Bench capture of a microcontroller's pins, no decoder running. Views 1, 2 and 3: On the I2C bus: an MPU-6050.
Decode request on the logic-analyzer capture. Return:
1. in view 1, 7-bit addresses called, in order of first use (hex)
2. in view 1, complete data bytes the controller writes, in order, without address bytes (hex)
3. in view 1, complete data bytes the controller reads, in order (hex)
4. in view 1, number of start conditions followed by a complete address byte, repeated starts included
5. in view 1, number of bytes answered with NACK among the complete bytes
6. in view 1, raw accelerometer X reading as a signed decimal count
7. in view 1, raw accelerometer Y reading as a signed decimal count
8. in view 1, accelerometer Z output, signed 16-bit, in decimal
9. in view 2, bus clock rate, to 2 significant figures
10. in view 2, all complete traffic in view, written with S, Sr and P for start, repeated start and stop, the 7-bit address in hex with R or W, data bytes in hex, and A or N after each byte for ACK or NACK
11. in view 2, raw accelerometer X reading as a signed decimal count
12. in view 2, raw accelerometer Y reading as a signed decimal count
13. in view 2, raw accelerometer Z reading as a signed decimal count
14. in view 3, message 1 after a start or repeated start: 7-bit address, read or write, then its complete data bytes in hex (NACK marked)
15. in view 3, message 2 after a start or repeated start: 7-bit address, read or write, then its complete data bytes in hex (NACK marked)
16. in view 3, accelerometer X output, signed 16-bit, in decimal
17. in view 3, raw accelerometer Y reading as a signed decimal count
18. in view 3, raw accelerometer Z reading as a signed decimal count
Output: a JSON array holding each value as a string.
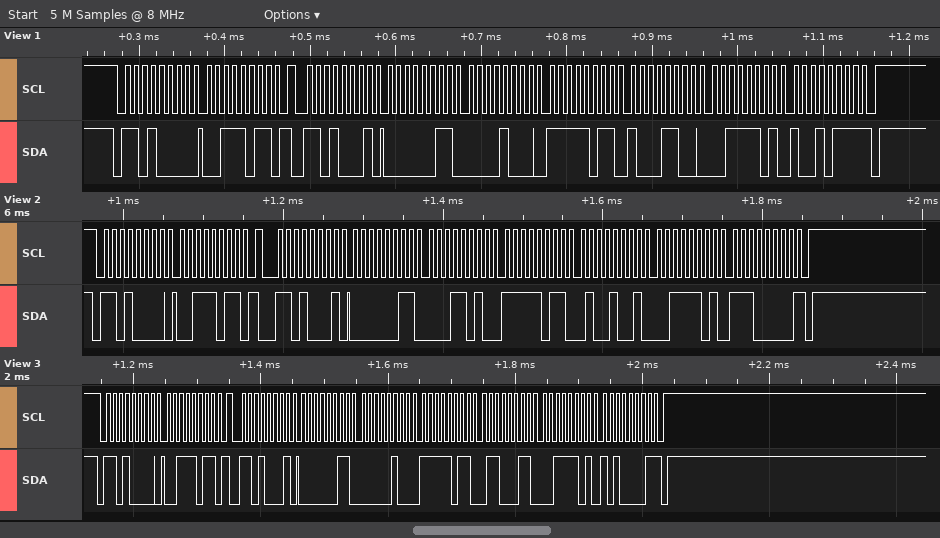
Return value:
["0x68", "3B", "03 08 FB 8C 3D 97", "2", "1", "776", "-1140", "15767", "100 kHz", "S 68W A 3B A Sr 68R A 03 A 1A A FB A 49 A 3D A E0 N P", "794", "-1207", "15840", "0x68 write: 3B", "0x68 read: 03 04 FB 63 3D A1 NACK", "772", "-1181", "15777"]
